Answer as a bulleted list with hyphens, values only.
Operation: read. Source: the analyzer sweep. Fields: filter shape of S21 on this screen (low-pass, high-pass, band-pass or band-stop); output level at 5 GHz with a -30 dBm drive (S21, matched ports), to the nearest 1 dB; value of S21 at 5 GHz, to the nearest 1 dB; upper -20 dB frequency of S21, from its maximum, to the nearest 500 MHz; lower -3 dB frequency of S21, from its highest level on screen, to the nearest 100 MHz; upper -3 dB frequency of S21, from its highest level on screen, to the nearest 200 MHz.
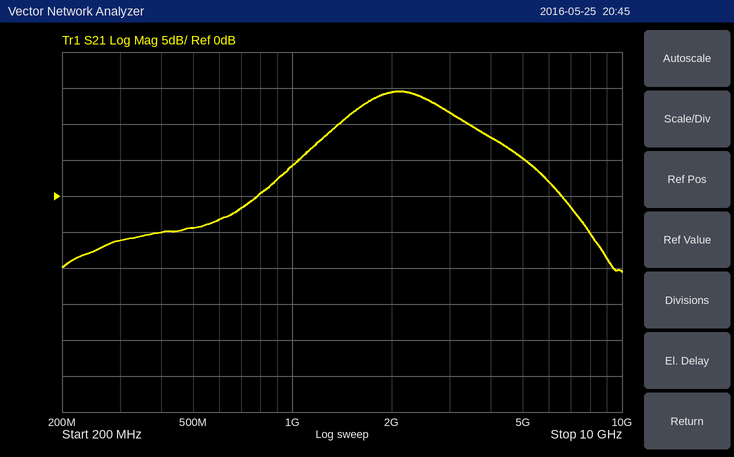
- band-pass
- -25 dBm
- 5 dB
- 8.0 GHz
- 1.5 GHz
- 3.0 GHz
